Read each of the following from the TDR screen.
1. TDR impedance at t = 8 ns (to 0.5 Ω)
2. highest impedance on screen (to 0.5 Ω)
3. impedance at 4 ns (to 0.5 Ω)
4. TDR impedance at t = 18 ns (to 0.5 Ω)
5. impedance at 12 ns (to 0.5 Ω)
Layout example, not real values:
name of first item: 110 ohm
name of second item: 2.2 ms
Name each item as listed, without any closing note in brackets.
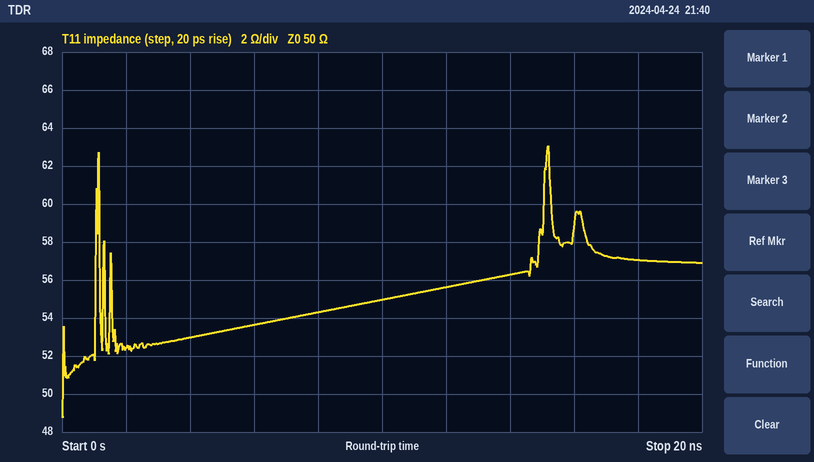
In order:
TDR impedance at t = 8 ns: 54.5 Ω
highest impedance on screen: 63.0 Ω
impedance at 4 ns: 53.0 Ω
TDR impedance at t = 18 ns: 57.0 Ω
impedance at 12 ns: 55.5 Ω
